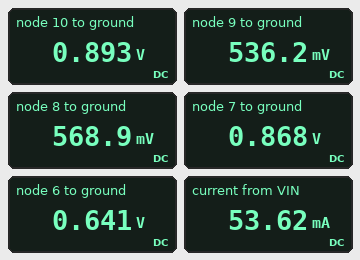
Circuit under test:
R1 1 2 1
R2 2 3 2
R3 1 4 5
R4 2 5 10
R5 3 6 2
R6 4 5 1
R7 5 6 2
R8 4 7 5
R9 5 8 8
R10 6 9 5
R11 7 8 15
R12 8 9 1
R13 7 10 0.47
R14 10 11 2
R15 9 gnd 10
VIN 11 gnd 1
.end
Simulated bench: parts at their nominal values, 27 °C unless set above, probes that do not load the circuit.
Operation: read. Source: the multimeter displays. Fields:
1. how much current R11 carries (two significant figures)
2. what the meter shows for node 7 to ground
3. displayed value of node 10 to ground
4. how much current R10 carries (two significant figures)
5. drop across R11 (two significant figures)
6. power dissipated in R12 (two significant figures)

20 mA
0.868 V
0.893 V
21 mA
300 mV
1.1 mW
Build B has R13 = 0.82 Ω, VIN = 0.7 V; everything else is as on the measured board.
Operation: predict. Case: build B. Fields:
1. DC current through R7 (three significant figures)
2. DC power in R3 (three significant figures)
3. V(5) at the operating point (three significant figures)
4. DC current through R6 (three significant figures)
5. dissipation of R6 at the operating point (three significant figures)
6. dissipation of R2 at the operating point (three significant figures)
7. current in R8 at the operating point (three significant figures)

10.2 mA
73.4 µW
461 mV
19.3 mA
374 µW
35.2 µW
23.2 mA
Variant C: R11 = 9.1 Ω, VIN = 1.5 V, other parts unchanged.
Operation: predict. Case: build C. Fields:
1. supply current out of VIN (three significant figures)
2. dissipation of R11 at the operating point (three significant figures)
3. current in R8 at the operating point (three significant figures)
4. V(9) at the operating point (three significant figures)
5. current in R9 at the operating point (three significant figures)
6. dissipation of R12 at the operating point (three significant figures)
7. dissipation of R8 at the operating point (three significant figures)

85.3 mA
15.8 mW
43.7 mA
853 mV
15.5 mA
3.26 mW
9.55 mW
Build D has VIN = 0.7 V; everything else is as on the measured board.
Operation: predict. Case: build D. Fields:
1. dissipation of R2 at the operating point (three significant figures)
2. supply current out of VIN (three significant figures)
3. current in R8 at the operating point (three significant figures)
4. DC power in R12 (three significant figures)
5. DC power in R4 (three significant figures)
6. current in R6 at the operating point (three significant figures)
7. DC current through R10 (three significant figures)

36.5 µW
37.5 mA
23.6 mA
522 µW
1.38 µW
19.7 mA
14.7 mA
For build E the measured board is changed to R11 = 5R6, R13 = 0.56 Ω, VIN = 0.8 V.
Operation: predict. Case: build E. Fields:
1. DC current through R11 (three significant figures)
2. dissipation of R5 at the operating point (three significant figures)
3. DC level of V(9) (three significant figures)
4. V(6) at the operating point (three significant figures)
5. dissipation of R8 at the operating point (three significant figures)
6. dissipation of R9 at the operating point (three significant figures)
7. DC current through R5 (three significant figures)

28.8 mA
27.5 µW
481 mV
546 mV
1.85 mW
303 µW
3.71 mA
